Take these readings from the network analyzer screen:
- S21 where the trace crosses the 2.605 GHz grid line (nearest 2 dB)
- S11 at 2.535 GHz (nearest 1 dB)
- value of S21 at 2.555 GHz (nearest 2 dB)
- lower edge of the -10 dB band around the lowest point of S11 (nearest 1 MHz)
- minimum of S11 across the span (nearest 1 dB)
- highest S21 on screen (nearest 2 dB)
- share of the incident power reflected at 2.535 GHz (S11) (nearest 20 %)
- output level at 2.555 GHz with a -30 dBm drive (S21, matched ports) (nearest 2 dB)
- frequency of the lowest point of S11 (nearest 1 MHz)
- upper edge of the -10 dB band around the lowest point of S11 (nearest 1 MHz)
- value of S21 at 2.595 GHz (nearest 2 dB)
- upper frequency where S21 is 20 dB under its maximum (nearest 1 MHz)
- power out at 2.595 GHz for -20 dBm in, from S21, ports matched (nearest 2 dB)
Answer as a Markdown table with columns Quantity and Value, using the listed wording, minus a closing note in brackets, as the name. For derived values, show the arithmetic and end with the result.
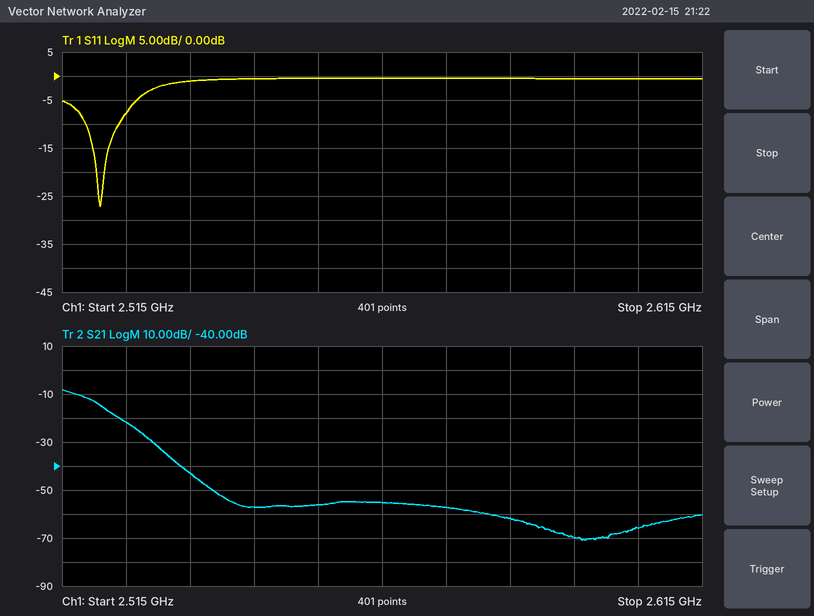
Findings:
| Quantity | Value |
|---|---|
| S21 where the trace crosses the 2.605 GHz grid line | -66 dB |
| S11 at 2.535 GHz | -1 dB |
| value of S21 at 2.555 GHz | -56 dB |
| lower edge of the -10 dB band around the lowest point of S11 | 2.519 GHz |
| minimum of S11 across the span | -27 dB |
| highest S21 on screen | -8 dB |
| share of the incident power reflected at 2.535 GHz (S11) | 10^(-1/10) ≈ 79.4 %, so 80 % to the nearest 20 % |
| output level at 2.555 GHz with a -30 dBm drive (S21, matched ports) | -30 dBm + (-56 dB) = -86 dBm |
| frequency of the lowest point of S11 | 2.521 GHz |
| upper edge of the -10 dB band around the lowest point of S11 | 2.524 GHz |
| value of S21 at 2.595 GHz | -70 dB |
| upper frequency where S21 is 20 dB under its maximum | 2.528 GHz |
| power out at 2.595 GHz for -20 dBm in, from S21, ports matched | -20 dBm + (-70 dB) = -90 dBm |
